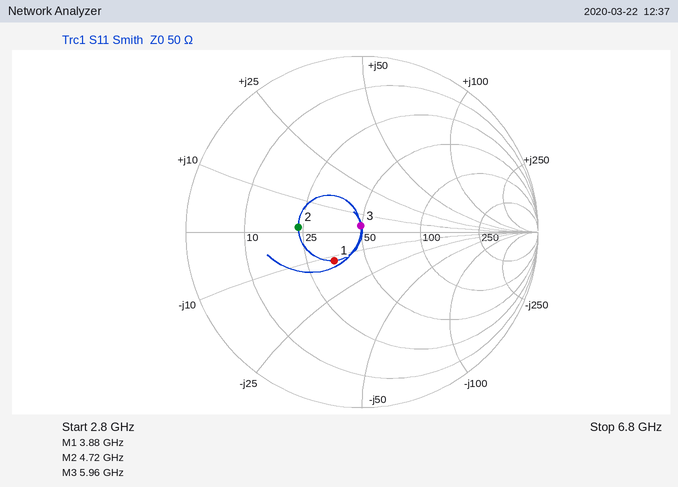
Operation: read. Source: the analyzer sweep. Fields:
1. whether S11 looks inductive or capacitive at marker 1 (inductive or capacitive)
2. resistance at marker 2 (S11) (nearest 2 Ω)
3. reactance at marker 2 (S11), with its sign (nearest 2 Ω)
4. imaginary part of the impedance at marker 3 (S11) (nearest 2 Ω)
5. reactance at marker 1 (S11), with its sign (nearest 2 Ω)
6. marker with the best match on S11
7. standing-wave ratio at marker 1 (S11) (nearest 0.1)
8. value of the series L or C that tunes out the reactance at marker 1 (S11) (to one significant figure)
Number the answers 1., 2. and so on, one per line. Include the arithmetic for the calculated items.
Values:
1. capacitive
2. 24 Ω
3. +2 Ω
4. +4 Ω
5. -12 Ω
6. marker 3
7. 1.6
8. L = 12 Ω/(2π × 3.88 GHz) ≈ 492 pH, so 500 pH to one significant figure
